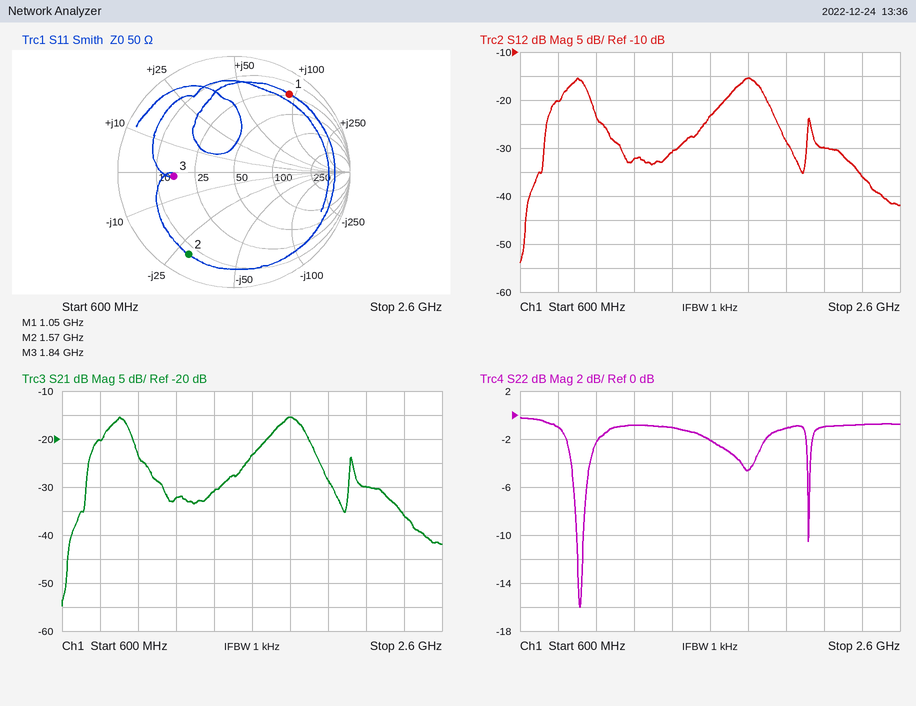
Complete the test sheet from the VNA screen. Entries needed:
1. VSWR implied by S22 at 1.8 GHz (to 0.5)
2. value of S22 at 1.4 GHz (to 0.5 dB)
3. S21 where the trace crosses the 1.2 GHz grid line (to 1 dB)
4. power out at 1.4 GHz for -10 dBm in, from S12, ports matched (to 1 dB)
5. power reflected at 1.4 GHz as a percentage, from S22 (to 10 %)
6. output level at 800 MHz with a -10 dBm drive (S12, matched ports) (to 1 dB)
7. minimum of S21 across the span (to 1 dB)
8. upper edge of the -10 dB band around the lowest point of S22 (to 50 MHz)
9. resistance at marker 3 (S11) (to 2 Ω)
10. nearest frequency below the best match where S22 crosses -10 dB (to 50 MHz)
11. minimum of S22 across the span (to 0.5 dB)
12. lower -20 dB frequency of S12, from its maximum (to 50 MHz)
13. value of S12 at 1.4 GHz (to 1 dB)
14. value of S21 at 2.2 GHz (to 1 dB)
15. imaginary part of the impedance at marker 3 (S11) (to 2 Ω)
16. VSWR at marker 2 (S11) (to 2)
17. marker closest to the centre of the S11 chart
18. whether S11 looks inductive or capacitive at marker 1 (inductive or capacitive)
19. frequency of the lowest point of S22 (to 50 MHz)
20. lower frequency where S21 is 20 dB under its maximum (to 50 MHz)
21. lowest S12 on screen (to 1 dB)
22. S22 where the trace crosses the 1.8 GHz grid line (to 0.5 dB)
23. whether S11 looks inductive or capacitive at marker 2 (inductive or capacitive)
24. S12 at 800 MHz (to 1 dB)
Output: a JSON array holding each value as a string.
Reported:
["4.0", "-1.0 dB", "-32 dB", "-41 dBm", "80 %", "-30 dBm", "-55 dB", "950 MHz", "16 Ω", "900 MHz", "-16.0 dB", "700 MHz", "-31 dB", "-30 dB", "-2 Ω", "10", "marker 3", "inductive", "900 MHz", "700 MHz", "-54 dB", "-4.5 dB", "capacitive", "-20 dB"]
